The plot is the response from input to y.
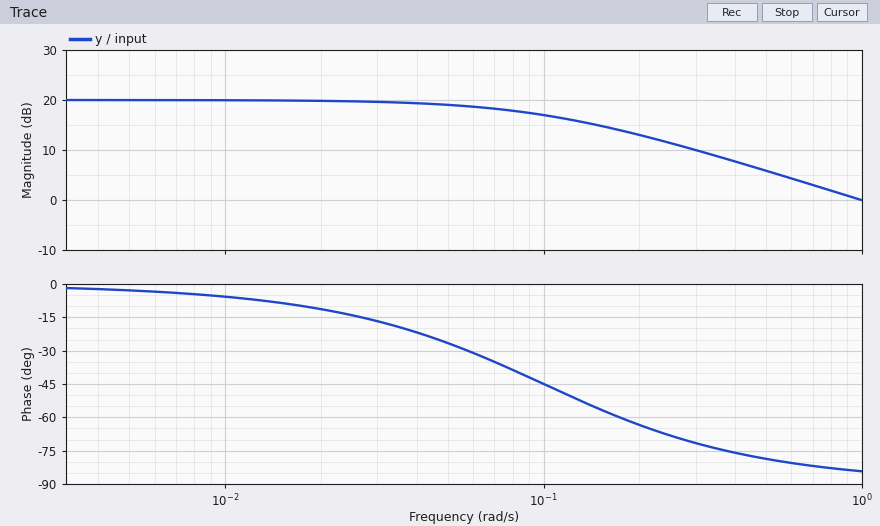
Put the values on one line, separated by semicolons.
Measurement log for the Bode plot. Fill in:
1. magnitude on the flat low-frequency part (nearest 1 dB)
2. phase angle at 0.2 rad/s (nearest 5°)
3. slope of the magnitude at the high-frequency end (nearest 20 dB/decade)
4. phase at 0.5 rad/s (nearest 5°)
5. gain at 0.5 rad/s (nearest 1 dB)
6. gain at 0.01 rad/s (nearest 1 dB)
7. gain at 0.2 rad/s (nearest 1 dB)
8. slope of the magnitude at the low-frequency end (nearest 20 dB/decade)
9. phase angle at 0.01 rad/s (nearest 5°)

20 dB; -65°; -20 dB/decade; -80°; 6 dB; 20 dB; 13 dB; 0 dB/decade; -5°
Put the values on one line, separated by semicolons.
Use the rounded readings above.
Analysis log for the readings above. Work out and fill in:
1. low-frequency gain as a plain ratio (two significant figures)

10
